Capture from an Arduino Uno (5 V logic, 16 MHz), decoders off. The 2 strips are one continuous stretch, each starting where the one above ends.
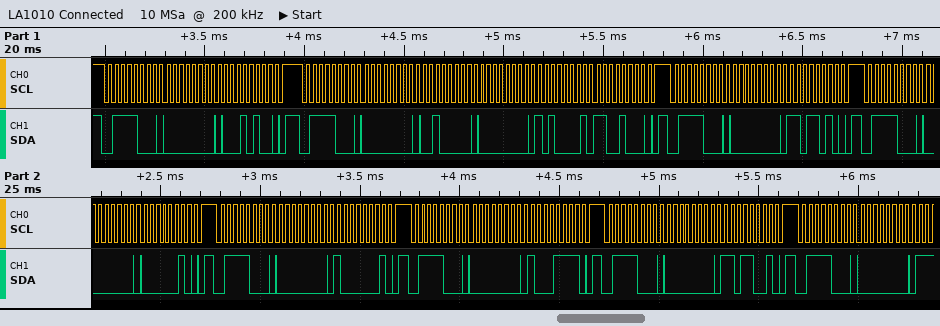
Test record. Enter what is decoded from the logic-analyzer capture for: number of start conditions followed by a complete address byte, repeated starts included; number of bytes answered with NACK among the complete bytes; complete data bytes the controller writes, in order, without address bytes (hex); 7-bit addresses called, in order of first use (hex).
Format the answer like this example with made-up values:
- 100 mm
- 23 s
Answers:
- 8
- 0
- 00 14 00 20 00 A1 C8 00 DA 00 02 00 81 00 8F 00 D9 00
- 0x3C
